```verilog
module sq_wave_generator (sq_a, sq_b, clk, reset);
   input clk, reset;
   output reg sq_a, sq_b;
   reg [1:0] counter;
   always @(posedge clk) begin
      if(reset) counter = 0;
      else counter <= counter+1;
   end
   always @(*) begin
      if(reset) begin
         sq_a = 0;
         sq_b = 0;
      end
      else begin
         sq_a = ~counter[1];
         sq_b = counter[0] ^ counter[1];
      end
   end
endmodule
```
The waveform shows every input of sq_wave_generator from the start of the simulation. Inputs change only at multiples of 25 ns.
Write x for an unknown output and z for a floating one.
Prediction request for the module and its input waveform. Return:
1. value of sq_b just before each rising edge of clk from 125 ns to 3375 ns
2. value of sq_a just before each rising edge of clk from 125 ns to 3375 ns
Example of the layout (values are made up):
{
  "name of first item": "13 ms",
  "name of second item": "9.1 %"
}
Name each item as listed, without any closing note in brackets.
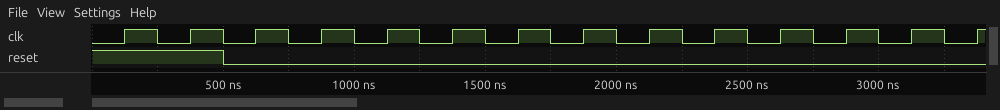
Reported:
{
  "value of sq_b just before each rising edge of clk from 125 ns to 3375 ns": "0 0 0 1 1 0 0 1 1 0 0 1 1 0",
  "value of sq_a just before each rising edge of clk from 125 ns to 3375 ns": "0 0 1 1 0 0 1 1 0 0 1 1 0 0"
}
